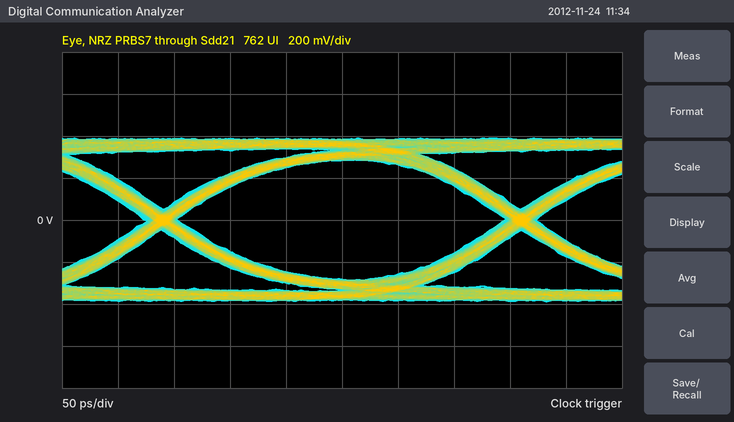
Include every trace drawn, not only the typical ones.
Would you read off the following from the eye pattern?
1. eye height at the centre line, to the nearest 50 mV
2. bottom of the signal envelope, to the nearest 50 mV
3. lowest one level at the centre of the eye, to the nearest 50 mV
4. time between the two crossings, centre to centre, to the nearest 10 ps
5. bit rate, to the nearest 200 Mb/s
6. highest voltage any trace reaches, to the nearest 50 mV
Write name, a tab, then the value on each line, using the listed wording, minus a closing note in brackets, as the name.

eye height at the centre line, to the nearest 50 mV	550 mV
bottom of the signal envelope, to the nearest 50 mV	-400 mV
lowest one level at the centre of the eye, to the nearest 50 mV	300 mV
time between the two crossings, centre to centre, to the nearest 10 ps	320 ps
bit rate, to the nearest 200 Mb/s	3.2 Gb/s
highest voltage any trace reaches, to the nearest 50 mV	400 mV
